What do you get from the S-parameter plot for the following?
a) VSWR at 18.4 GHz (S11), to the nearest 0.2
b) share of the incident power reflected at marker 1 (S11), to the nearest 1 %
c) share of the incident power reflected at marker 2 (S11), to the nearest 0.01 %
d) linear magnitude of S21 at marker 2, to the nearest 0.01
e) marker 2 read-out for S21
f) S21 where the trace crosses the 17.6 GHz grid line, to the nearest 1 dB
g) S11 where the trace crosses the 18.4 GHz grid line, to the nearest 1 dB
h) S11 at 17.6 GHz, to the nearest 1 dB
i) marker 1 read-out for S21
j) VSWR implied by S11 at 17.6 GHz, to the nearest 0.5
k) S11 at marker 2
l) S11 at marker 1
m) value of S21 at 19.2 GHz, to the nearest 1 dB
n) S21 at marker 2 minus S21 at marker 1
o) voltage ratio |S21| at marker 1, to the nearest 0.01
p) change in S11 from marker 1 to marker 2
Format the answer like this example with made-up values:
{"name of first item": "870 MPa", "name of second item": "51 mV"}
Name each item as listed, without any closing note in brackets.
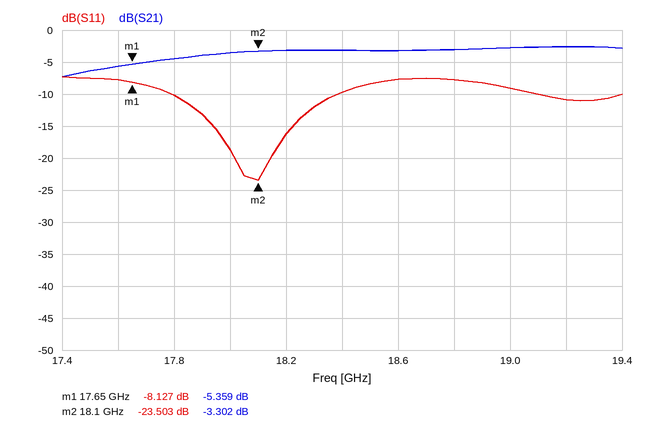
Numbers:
{"VSWR at 18.4 GHz (S11), to the nearest 0.2": "2.0", "share of the incident power reflected at marker 1 (S11), to the nearest 1 %": "15 %", "share of the incident power reflected at marker 2 (S11), to the nearest 0.01 %": "0.45 %", "linear magnitude of S21 at marker 2, to the nearest 0.01": "0.68", "marker 2 read-out for S21": "-3.302 dB", "S21 where the trace crosses the 17.6 GHz grid line, to the nearest 1 dB": "-6 dB", "S11 where the trace crosses the 18.4 GHz grid line, to the nearest 1 dB": "-10 dB", "S11 at 17.6 GHz, to the nearest 1 dB": "-8 dB", "marker 1 read-out for S21": "-5.359 dB", "VSWR implied by S11 at 17.6 GHz, to the nearest 0.5": "2.5", "S11 at marker 2": "-23.503 dB", "S11 at marker 1": "-8.127 dB", "value of S21 at 19.2 GHz, to the nearest 1 dB": "-3 dB", "S21 at marker 2 minus S21 at marker 1": "2.057 dB", "voltage ratio |S21| at marker 1, to the nearest 0.01": "0.54", "change in S11 from marker 1 to marker 2": "-15.376 dB"}
